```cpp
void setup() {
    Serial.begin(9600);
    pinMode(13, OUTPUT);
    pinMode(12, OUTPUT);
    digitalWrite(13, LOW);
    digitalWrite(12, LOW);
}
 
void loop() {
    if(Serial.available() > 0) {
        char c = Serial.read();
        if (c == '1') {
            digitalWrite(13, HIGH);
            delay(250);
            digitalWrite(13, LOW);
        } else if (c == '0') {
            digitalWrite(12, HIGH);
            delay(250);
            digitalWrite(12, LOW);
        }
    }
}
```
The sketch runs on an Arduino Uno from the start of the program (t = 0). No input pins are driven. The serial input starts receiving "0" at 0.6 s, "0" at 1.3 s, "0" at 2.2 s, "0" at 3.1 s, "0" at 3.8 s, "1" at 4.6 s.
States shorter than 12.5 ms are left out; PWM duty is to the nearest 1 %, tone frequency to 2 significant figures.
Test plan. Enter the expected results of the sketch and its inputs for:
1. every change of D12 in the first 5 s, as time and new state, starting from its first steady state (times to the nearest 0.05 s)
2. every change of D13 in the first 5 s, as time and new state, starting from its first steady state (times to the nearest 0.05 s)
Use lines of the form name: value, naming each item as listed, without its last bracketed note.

every change of D12 in the first 5 s, as time and new state, starting from its first steady state: 0 s low; 0.6 s high; 0.85 s low; 1.3 s high; 1.55 s low; 2.2 s high; 2.45 s low; 3.1 s high; 3.35 s low; 3.8 s high; 4.05 s low
every change of D13 in the first 5 s, as time and new state, starting from its first steady state: 0 s low; 4.6 s high; 4.85 s low
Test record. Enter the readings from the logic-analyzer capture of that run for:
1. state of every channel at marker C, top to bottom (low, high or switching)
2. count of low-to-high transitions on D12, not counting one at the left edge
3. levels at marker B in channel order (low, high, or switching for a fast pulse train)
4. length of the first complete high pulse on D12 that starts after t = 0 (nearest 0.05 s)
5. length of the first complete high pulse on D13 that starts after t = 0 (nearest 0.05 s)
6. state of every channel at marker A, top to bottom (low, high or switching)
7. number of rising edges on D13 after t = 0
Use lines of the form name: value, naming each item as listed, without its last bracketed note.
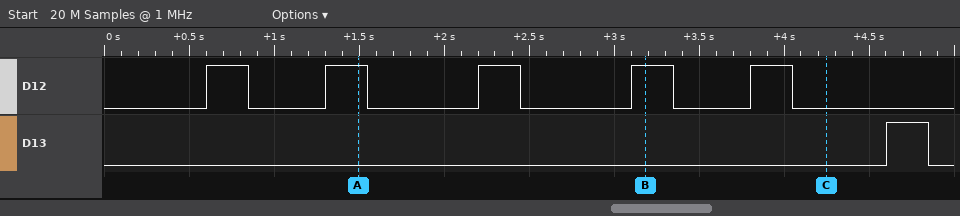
state of every channel at marker C, top to bottom: D12 low, D13 low
count of low-to-high transitions on D12, not counting one at the left edge: 5
levels at marker B in channel order: D12 high, D13 low
length of the first complete high pulse on D12 that starts after t = 0: 0.25 s
length of the first complete high pulse on D13 that starts after t = 0: 0.25 s
state of every channel at marker A, top to bottom: D12 high, D13 low
number of rising edges on D13 after t = 0: 1
